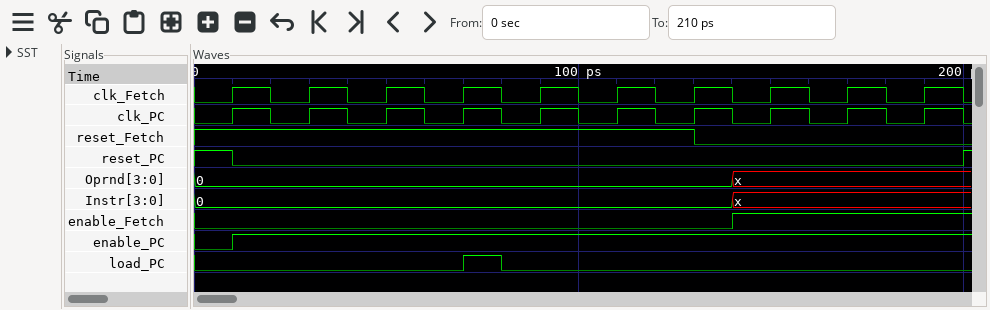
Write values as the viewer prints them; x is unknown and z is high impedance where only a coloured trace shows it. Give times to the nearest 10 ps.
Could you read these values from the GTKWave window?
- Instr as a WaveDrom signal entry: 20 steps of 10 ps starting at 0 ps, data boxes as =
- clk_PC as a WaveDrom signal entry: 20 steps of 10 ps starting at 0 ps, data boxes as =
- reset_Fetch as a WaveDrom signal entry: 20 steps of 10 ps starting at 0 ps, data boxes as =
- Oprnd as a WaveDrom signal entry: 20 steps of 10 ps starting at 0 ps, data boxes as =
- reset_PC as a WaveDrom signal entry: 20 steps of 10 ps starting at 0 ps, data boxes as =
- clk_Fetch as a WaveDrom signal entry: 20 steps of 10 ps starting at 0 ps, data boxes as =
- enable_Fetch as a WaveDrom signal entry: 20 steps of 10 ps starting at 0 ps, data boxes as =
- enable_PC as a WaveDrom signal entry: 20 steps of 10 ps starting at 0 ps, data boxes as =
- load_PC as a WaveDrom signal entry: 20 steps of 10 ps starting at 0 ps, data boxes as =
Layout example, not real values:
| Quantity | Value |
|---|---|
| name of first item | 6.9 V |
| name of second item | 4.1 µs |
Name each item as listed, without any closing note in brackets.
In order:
| Quantity | Value |
|---|---|
| Instr as a WaveDrom signal entry: 20 steps of 10 ps starting at 0 ps, data boxes as = | {name: 'Instr', wave: '=.............x.....', data: '0'} |
| clk_PC as a WaveDrom signal entry: 20 steps of 10 ps starting at 0 ps, data boxes as = | {name: 'clk_PC', wave: '01010101010101010101'} |
| reset_Fetch as a WaveDrom signal entry: 20 steps of 10 ps starting at 0 ps, data boxes as = | {name: 'reset_Fetch', wave: '1............0......'} |
| Oprnd as a WaveDrom signal entry: 20 steps of 10 ps starting at 0 ps, data boxes as = | {name: 'Oprnd', wave: '=.............x.....', data: '0'} |
| reset_PC as a WaveDrom signal entry: 20 steps of 10 ps starting at 0 ps, data boxes as = | {name: 'reset_PC', wave: '10..................'} |
| clk_Fetch as a WaveDrom signal entry: 20 steps of 10 ps starting at 0 ps, data boxes as = | {name: 'clk_Fetch', wave: '01010101010101010101'} |
| enable_Fetch as a WaveDrom signal entry: 20 steps of 10 ps starting at 0 ps, data boxes as = | {name: 'enable_Fetch', wave: '0.............1.....'} |
| enable_PC as a WaveDrom signal entry: 20 steps of 10 ps starting at 0 ps, data boxes as = | {name: 'enable_PC', wave: '01..................'} |
| load_PC as a WaveDrom signal entry: 20 steps of 10 ps starting at 0 ps, data boxes as = | {name: 'load_PC', wave: '0......10...........'} |
